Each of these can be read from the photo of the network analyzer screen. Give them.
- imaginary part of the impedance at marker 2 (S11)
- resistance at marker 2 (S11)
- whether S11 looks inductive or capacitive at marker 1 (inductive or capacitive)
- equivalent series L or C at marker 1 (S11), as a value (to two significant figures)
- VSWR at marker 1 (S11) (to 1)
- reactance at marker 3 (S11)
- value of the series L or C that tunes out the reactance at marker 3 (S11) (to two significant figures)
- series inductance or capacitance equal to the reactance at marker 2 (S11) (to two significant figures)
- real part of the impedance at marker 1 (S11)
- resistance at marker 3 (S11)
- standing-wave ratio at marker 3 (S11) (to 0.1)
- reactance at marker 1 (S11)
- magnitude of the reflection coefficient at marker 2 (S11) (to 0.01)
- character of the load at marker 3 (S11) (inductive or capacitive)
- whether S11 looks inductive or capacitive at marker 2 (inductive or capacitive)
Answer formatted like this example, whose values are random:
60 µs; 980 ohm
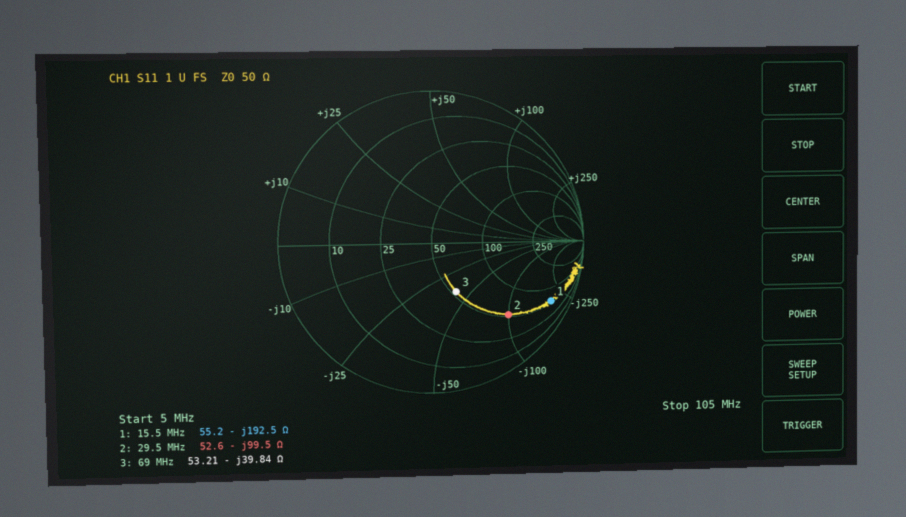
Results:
-99.5 Ω; 52.6 Ω; capacitive; 53 pF; 15; -39.84 Ω; 92 nH; 54 pF; 55.2 Ω; 53.21 Ω; 2.1; -192.5 Ω; 0.70; capacitive; capacitive
